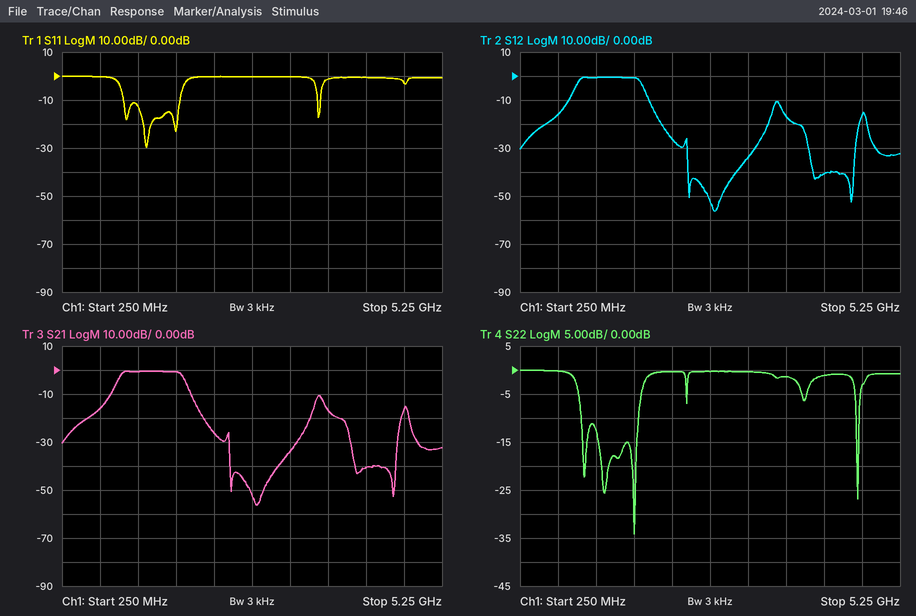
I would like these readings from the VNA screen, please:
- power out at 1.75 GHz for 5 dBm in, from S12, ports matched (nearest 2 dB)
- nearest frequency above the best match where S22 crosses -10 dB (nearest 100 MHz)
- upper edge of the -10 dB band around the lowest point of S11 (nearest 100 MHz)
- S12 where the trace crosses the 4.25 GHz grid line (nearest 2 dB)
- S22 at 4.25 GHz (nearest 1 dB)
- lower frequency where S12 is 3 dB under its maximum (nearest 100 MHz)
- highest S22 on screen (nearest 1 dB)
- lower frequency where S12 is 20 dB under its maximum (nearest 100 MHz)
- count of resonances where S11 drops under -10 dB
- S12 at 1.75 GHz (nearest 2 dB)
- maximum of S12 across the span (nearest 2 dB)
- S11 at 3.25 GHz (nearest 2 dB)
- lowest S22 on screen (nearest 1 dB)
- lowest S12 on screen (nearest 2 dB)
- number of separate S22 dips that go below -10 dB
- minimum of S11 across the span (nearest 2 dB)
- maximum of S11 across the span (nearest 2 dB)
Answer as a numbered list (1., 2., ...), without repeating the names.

1. 4 dBm
2. 1.8 GHz
3. 1.8 GHz
4. -40 dB
5. -1 dB
6. 1.0 GHz
7. 0 dB
8. 600 MHz
9. 4
10. 0 dB
11. 0 dB
12. 0 dB
13. -34 dB
14. -56 dB
15. 4
16. -30 dB
17. 0 dB
